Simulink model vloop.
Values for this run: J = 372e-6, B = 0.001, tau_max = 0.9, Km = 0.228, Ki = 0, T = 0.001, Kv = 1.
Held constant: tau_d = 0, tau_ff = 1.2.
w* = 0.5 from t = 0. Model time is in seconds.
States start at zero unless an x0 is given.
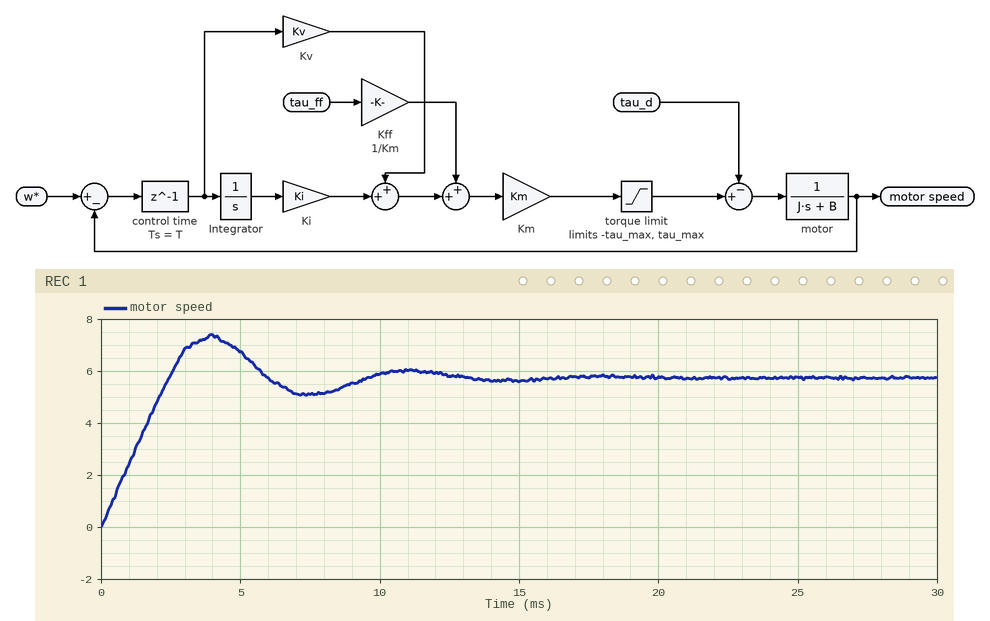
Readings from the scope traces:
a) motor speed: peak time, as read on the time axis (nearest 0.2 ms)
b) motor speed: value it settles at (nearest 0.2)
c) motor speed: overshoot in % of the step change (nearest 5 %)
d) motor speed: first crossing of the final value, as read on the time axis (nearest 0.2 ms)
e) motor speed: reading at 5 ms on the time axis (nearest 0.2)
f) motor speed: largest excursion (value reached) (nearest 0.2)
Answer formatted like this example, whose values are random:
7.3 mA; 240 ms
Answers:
4.0 ms; 5.8; 30 %; 2.4 ms; 6.8; 7.4
